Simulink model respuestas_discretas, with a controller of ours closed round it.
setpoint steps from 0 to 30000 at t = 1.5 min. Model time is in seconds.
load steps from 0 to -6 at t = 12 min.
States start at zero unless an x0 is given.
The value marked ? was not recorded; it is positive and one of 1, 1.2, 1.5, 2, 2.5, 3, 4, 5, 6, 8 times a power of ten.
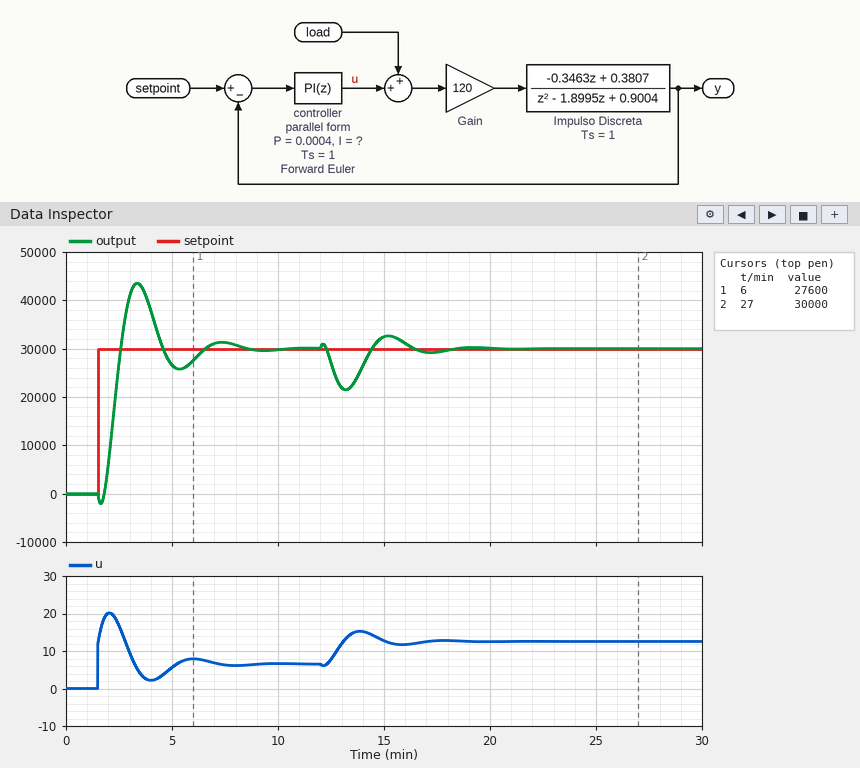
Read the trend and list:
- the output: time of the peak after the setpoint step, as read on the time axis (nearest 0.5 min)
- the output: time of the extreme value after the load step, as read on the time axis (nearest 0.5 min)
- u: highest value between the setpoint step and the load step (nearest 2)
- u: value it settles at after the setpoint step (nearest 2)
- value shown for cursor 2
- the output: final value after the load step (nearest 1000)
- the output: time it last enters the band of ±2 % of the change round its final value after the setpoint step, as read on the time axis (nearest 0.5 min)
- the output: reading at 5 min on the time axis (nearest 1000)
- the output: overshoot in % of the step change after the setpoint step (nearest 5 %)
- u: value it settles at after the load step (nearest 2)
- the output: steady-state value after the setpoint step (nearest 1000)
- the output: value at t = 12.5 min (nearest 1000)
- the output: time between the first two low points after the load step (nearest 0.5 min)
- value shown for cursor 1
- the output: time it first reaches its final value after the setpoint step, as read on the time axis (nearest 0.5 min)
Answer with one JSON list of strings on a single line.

["3.5 min", "13.0 min", "20", "6", "30000", "30000", "8.0 min", "27000", "45 %", "12", "30000", "27000", "4.0 min", "27600", "2.5 min"]
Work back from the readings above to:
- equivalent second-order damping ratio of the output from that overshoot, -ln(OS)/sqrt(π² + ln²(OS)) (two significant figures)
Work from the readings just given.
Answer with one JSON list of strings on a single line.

["0.25"]
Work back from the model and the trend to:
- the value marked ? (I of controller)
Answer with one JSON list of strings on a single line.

["1.2e-05"]
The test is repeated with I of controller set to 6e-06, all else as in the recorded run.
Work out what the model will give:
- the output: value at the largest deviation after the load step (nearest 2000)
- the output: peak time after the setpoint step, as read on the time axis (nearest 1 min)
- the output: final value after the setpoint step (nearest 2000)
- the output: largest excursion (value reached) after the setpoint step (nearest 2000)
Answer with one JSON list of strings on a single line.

["22000", "4 min", "30000", "34000"]
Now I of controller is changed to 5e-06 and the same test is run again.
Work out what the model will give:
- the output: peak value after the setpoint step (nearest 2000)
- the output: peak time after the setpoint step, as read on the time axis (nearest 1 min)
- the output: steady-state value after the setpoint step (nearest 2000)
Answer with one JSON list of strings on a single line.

["32000", "4 min", "30000"]
